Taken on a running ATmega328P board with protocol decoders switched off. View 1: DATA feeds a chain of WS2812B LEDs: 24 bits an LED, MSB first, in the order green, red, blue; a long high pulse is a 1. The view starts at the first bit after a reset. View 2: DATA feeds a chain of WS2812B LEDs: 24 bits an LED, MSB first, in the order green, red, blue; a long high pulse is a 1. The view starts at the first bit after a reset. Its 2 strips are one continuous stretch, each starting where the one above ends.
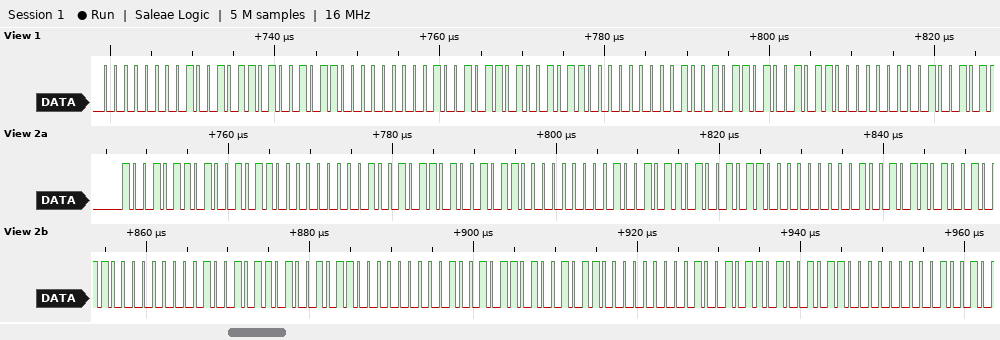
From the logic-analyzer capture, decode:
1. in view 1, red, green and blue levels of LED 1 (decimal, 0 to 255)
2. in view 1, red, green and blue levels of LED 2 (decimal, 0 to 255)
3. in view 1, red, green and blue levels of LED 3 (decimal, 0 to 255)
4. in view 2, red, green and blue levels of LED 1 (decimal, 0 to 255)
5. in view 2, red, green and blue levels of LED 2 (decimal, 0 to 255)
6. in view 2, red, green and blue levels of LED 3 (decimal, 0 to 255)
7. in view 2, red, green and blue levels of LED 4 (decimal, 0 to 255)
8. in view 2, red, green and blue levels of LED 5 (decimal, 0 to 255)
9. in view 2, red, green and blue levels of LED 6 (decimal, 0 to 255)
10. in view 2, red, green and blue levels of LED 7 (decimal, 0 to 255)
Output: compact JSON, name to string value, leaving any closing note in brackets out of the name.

{"in view 1, red, green and blue levels of LED 1": "150, 0, 150", "in view 1, red, green and blue levels of LED 2": "150, 0, 150", "in view 1, red, green and blue levels of LED 3": "150, 0, 150", "in view 2, red, green and blue levels of LED 1": "150, 150, 0", "in view 2, red, green and blue levels of LED 2": "150, 150, 0", "in view 2, red, green and blue levels of LED 3": "150, 150, 0", "in view 2, red, green and blue levels of LED 4": "150, 150, 0", "in view 2, red, green and blue levels of LED 5": "150, 150, 0", "in view 2, red, green and blue levels of LED 6": "150, 150, 0", "in view 2, red, green and blue levels of LED 7": "150, 150, 0"}
